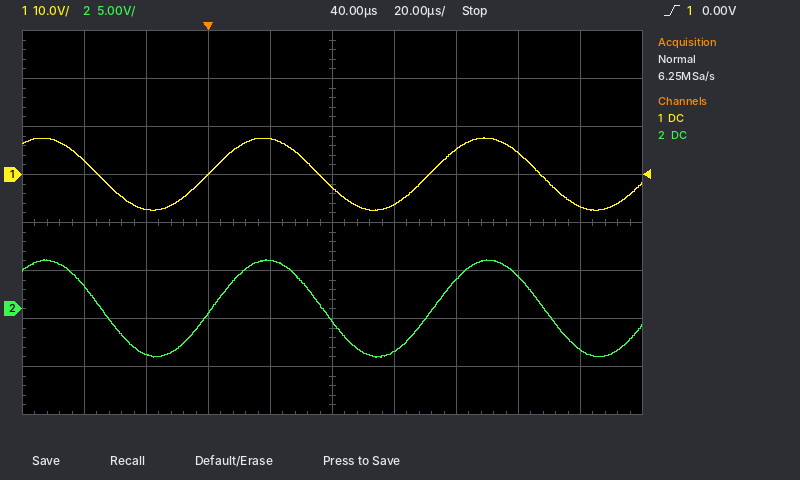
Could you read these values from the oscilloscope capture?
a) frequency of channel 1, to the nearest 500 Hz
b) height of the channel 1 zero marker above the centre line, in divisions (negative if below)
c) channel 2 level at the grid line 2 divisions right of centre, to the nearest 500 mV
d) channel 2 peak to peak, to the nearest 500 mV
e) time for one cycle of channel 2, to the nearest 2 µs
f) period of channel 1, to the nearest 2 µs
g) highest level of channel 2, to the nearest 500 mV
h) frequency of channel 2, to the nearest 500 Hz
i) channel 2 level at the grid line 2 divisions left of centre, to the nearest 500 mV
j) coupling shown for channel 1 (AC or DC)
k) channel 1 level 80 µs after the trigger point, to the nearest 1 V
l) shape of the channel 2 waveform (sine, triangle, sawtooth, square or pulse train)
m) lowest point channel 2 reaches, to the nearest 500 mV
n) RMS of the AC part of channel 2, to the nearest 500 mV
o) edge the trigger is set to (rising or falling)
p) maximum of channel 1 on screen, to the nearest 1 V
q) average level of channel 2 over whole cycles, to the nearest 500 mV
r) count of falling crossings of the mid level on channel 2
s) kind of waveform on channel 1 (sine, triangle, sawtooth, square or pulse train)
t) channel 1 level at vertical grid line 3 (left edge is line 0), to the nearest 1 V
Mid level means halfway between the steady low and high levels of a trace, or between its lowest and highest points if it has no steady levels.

14.0 kHz
+1.0 div
3.0 V
10.0 V
72 µs
72 µs
5.0 V
14.0 kHz
-500 mV
DC
5 V
sine
-5.0 V
3.5 V
rising
8 V
0.0 V
3
sine
0 V
